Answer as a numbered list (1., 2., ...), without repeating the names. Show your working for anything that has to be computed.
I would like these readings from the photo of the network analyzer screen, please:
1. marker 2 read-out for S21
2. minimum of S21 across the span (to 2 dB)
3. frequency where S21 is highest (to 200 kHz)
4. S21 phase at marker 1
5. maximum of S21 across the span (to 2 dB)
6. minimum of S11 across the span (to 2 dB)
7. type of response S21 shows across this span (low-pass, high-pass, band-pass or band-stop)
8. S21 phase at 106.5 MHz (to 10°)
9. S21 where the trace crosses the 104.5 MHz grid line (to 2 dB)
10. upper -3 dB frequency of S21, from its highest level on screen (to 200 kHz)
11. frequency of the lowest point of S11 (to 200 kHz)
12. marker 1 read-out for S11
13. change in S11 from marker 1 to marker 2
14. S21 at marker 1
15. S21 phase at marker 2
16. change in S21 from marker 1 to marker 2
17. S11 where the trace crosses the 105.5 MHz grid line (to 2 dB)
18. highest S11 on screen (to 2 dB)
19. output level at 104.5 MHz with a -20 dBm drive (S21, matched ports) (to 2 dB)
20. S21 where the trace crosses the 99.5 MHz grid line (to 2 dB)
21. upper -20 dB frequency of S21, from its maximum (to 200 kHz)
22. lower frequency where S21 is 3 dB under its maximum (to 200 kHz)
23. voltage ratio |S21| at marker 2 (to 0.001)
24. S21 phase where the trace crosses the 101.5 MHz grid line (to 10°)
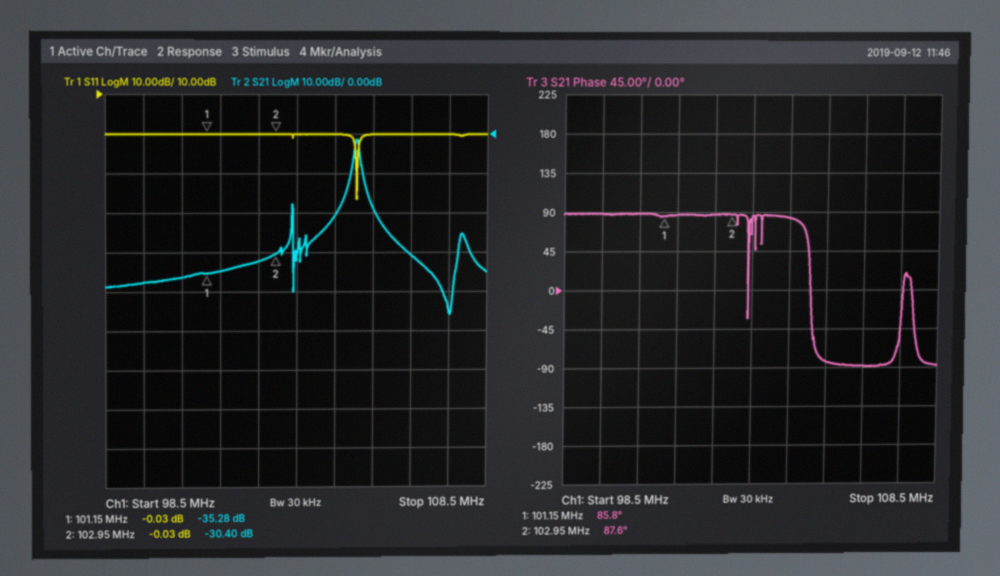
1. -30.40 dB
2. -46 dB
3. 105.0 MHz
4. 85.8°
5. -2 dB
6. -16 dB
7. band-pass
8. -90°
9. -20 dB
10. 105.2 MHz
11. 105.0 MHz
12. -0.03 dB
13. -0.03 − (-0.03) = 0.00 dB
14. -35.28 dB
15. 87.6°
16. -30.4 − (-35.28) = 4.88 dB
17. 0 dB
18. 0 dB
19. -20 dBm + (-20 dB) = -40 dBm
20. -38 dB
21. 105.6 MHz
22. 105.0 MHz
23. 10^(-30.4/20) ≈ 0.030
24. 90°
